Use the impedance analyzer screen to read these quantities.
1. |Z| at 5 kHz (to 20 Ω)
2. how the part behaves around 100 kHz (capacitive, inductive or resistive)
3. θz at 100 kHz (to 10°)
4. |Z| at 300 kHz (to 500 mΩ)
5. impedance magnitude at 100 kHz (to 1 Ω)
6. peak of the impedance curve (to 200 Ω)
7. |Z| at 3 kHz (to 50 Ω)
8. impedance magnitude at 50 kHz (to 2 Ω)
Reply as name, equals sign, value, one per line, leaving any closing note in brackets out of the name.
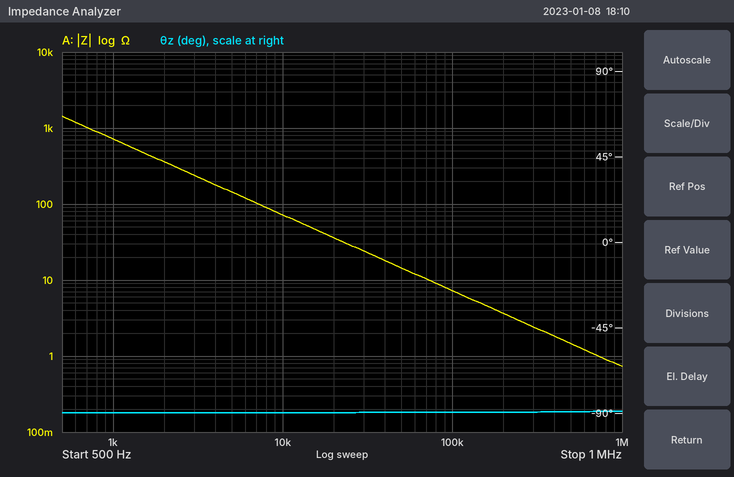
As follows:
|Z| at 5 kHz = 140 Ω
how the part behaves around 100 kHz = capacitive
θz at 100 kHz = -90°
|Z| at 300 kHz = 2.5 Ω
impedance magnitude at 100 kHz = 7 Ω
peak of the impedance curve = 1.4 kΩ
|Z| at 3 kHz = 250 Ω
impedance magnitude at 50 kHz = 14 Ω
